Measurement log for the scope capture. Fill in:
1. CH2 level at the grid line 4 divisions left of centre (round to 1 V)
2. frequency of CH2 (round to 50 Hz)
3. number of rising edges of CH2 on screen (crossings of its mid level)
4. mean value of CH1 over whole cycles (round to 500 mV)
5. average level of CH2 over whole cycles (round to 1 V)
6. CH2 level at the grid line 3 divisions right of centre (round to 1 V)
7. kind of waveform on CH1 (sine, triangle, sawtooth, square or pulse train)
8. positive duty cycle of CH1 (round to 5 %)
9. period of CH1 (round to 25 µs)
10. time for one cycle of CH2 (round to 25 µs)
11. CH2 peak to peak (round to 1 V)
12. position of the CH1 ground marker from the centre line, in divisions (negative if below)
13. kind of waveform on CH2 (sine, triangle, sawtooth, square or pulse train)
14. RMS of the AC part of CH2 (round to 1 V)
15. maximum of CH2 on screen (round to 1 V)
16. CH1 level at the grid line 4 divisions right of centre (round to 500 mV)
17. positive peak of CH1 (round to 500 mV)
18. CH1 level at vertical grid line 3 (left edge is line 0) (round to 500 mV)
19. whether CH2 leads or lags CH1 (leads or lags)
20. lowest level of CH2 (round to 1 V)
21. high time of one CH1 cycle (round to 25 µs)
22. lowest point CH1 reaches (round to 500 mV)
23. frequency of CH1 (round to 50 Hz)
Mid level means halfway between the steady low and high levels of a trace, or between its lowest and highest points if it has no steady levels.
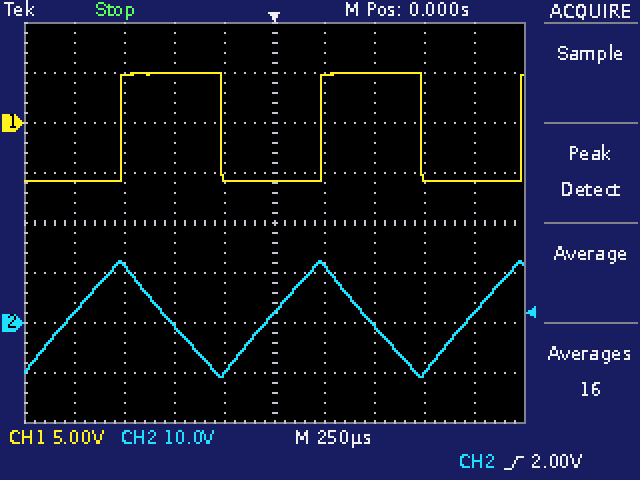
2 V
1.00 kHz
3
-500 mV
1 V
-10 V
square
50 %
1.000 ms
1.000 ms
23 V
+2.0 div
triangle
7 V
12 V
-6.0 V
5.0 V
5.0 V
leads
-11 V
500 µs
-6.0 V
1.00 kHz
